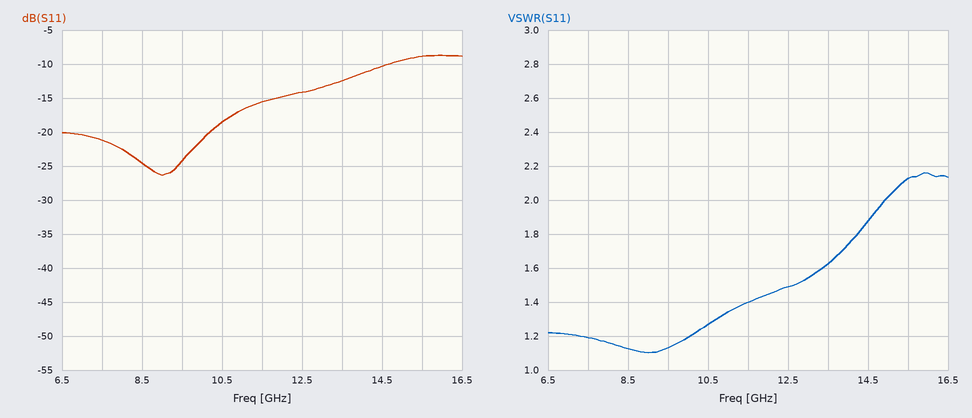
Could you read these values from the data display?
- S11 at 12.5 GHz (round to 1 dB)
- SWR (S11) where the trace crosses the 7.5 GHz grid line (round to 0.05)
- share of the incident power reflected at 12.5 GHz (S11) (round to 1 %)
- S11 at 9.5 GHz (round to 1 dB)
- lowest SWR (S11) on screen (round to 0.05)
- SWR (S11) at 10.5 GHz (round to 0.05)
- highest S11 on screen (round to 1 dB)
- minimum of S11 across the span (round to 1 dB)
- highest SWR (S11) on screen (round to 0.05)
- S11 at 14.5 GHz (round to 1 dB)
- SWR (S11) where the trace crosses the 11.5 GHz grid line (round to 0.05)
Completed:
-14 dB
1.20
4 %
-24 dB
1.10
1.25
-9 dB
-26 dB
2.15
-10 dB
1.40
